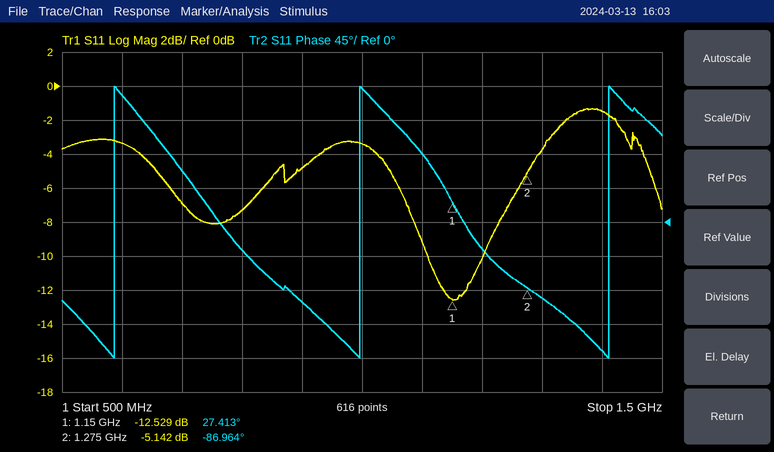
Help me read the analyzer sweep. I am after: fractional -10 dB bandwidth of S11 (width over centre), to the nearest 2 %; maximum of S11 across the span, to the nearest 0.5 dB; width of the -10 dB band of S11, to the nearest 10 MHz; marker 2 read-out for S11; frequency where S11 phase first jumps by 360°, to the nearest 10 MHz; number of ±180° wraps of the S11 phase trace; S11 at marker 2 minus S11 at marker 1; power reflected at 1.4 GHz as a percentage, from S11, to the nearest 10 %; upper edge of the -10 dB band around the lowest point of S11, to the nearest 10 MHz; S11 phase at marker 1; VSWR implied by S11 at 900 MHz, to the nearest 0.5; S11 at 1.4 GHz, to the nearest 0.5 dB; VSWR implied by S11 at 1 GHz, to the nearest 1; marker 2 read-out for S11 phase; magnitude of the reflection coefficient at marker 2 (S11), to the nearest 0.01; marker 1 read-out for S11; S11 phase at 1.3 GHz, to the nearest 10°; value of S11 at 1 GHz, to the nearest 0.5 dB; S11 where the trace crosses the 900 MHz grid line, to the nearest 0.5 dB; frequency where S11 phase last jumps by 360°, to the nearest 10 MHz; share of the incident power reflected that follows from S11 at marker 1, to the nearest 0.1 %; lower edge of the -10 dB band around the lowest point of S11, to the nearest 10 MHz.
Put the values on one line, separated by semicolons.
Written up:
8 %; -1.5 dB; 90 MHz; -5.142 dB; 590 MHz; 3; 7.387 dB; 70 %; 1.20 GHz; 27.413°; 3.5; -1.5 dB; 5; -86.964°; 0.55; -12.529 dB; -100°; -3.5 dB; -5.0 dB; 1.41 GHz; 5.6 %; 1.11 GHz
